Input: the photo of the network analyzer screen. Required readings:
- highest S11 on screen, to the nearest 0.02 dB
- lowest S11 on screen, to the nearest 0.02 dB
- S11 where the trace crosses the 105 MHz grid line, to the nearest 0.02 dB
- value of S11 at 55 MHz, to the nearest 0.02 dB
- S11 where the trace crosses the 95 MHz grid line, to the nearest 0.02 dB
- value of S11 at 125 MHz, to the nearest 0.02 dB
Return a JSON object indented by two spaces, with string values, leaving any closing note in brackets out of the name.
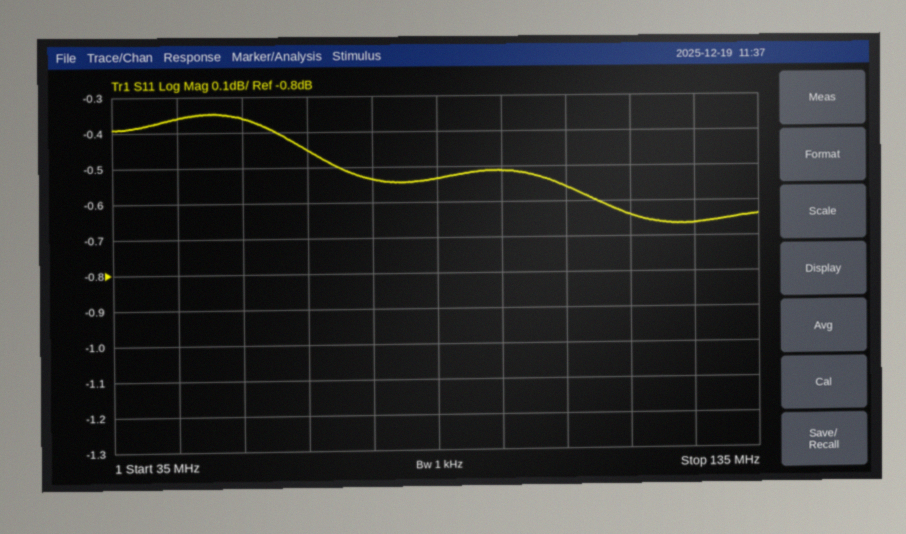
{
  "highest S11 on screen, to the nearest 0.02 dB": "-0.34 dB",
  "lowest S11 on screen, to the nearest 0.02 dB": "-0.66 dB",
  "S11 where the trace crosses the 105 MHz grid line, to the nearest 0.02 dB": "-0.56 dB",
  "value of S11 at 55 MHz, to the nearest 0.02 dB": "-0.36 dB",
  "S11 where the trace crosses the 95 MHz grid line, to the nearest 0.02 dB": "-0.52 dB",
  "value of S11 at 125 MHz, to the nearest 0.02 dB": "-0.66 dB"
}
